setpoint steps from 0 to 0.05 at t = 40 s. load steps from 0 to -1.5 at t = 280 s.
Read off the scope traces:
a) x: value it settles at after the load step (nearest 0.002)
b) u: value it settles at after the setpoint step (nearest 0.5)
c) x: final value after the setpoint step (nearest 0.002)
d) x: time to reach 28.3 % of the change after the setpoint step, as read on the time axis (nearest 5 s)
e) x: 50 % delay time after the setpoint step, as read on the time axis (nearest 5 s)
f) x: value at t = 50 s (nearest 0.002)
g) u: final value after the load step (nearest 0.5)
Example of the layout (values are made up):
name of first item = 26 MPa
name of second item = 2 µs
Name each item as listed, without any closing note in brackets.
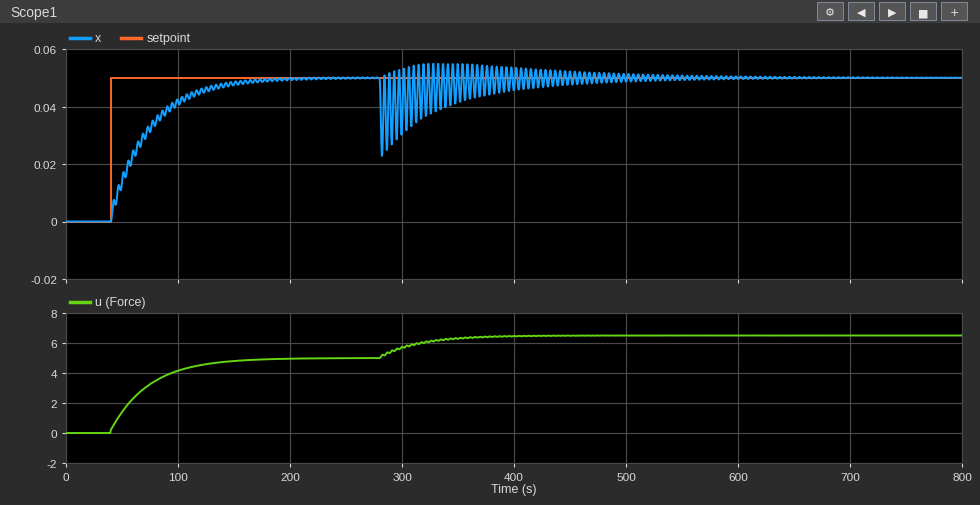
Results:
x: value it settles at after the load step = 0.050
u: value it settles at after the setpoint step = 5.0
x: final value after the setpoint step = 0.050
x: time to reach 28.3 % of the change after the setpoint step, as read on the time axis = 50 s
x: 50 % delay time after the setpoint step, as read on the time axis = 65 s
x: value at t = 50 s = 0.014
u: final value after the load step = 6.5
